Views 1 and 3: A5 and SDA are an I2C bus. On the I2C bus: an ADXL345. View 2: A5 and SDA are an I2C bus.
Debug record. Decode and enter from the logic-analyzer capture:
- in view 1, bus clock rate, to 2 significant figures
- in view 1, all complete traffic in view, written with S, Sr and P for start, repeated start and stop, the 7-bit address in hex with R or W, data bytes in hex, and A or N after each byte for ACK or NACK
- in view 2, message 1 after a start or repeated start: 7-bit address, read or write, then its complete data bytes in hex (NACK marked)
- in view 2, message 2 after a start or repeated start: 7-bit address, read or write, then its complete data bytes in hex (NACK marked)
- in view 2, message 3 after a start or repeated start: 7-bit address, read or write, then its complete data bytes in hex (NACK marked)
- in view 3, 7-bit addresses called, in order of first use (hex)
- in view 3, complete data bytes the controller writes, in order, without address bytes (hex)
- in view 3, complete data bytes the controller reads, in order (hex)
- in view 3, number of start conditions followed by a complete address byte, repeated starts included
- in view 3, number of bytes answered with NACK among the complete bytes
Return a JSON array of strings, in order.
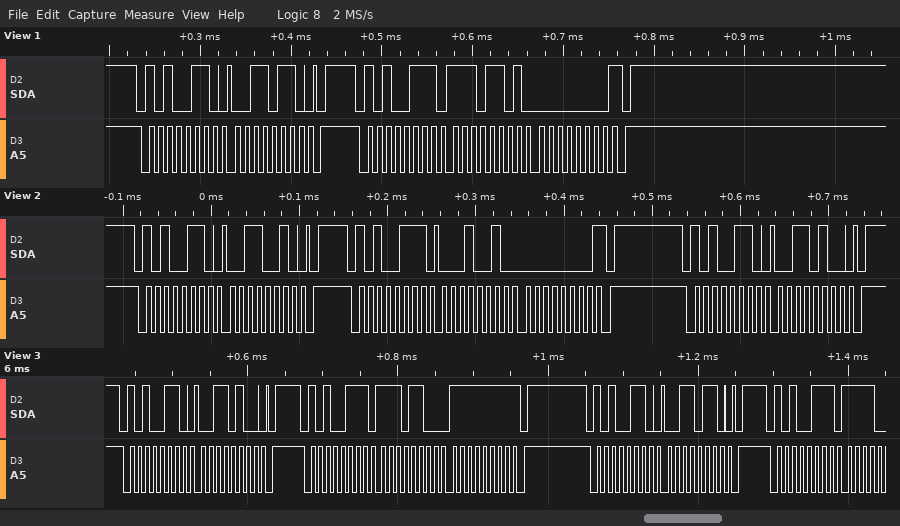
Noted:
["100 kHz", "S 53W A 36 A P S 53R A ED A 00 N P", "0x53 write: 32", "0x53 read: 12 00 NACK", "0x53 write: 34", "0x53", "34 36", "EC FF", "4", "1"]
